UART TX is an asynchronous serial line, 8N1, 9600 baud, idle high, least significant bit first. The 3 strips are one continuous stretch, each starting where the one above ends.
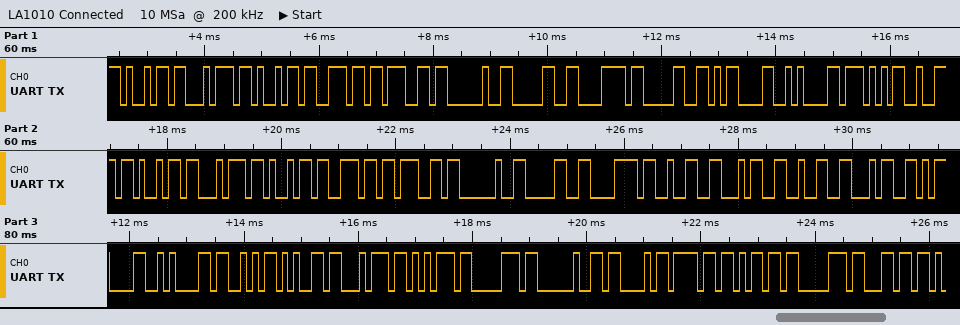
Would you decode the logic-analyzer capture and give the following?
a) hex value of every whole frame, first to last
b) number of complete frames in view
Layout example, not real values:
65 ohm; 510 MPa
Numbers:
69 74 69 6E 67 20 30 78 30 0D 0A 57 72 69 74 69 6E 67 20 30 78 32 34 32 34 0D 0A 53 65 74 75 70 20 43 6F 6D 70 6C; 38
